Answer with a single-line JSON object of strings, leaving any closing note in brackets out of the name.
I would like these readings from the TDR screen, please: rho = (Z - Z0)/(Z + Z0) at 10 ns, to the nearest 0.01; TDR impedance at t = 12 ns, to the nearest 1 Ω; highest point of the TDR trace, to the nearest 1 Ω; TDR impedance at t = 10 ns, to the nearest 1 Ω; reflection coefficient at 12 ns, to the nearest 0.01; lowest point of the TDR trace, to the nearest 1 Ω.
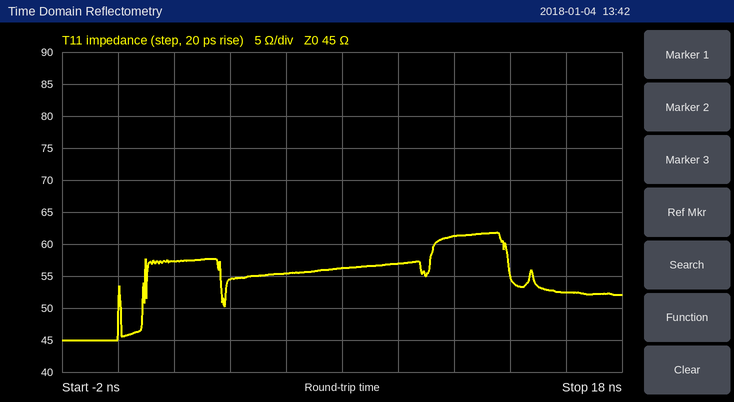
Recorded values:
{"rho = (Z - Z0)/(Z + Z0) at 10 ns, to the nearest 0.01": "+0.12", "TDR impedance at t = 12 ns, to the nearest 1 Ω": "61 Ω", "highest point of the TDR trace, to the nearest 1 Ω": "62 Ω", "TDR impedance at t = 10 ns, to the nearest 1 Ω": "57 Ω", "reflection coefficient at 12 ns, to the nearest 0.01": "+0.15", "lowest point of the TDR trace, to the nearest 1 Ω": "45 Ω"}
